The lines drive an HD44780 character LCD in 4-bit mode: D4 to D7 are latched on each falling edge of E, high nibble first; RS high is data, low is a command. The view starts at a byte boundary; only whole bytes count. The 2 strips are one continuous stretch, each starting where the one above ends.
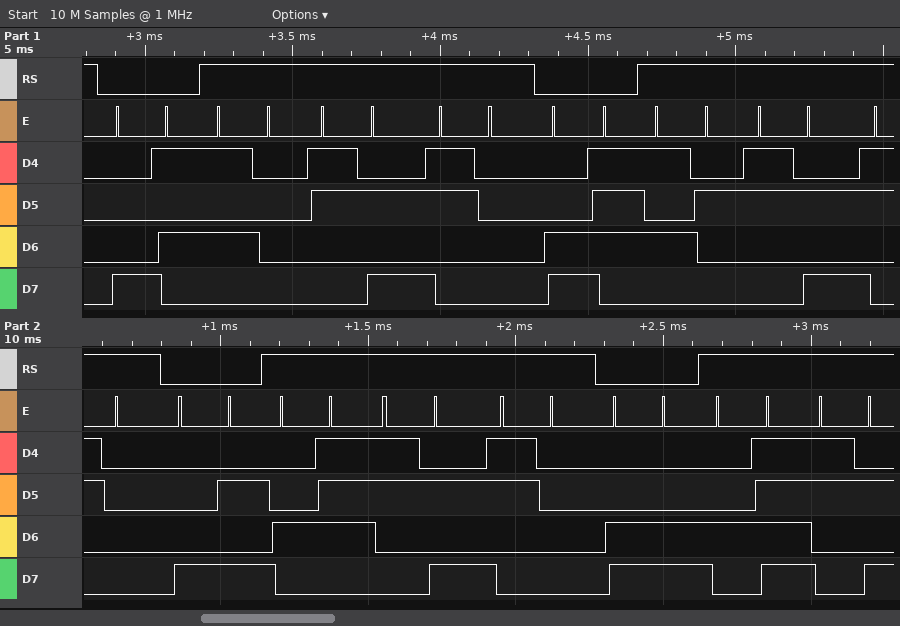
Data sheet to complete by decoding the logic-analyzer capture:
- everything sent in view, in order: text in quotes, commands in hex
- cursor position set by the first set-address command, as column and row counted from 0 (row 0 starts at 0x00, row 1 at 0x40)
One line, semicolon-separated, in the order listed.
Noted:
0x85 "P:0" 0xC7 "R:0" 0x8A "G:0" 0xCC "O:"; column 5, row 0
